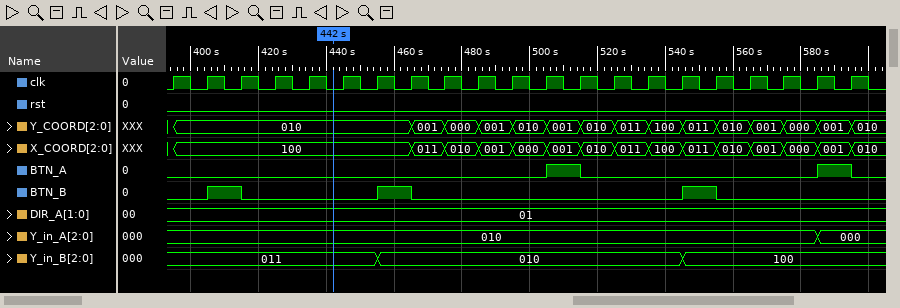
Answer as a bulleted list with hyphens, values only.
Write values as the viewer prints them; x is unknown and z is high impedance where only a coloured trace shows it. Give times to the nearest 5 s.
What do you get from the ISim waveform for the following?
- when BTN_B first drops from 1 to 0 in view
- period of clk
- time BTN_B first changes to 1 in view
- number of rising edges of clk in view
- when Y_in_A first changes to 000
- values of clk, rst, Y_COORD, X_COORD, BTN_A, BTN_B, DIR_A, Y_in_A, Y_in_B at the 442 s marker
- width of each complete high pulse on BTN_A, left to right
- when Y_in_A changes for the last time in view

- 415 s
- 10 s
- 405 s
- 21
- 585 s
- clk=0, rst=0, Y_COORD=010, X_COORD=100, BTN_A=0, BTN_B=0, DIR_A=01, Y_in_A=010, Y_in_B=011
- 10 s, 10 s
- 585 s
